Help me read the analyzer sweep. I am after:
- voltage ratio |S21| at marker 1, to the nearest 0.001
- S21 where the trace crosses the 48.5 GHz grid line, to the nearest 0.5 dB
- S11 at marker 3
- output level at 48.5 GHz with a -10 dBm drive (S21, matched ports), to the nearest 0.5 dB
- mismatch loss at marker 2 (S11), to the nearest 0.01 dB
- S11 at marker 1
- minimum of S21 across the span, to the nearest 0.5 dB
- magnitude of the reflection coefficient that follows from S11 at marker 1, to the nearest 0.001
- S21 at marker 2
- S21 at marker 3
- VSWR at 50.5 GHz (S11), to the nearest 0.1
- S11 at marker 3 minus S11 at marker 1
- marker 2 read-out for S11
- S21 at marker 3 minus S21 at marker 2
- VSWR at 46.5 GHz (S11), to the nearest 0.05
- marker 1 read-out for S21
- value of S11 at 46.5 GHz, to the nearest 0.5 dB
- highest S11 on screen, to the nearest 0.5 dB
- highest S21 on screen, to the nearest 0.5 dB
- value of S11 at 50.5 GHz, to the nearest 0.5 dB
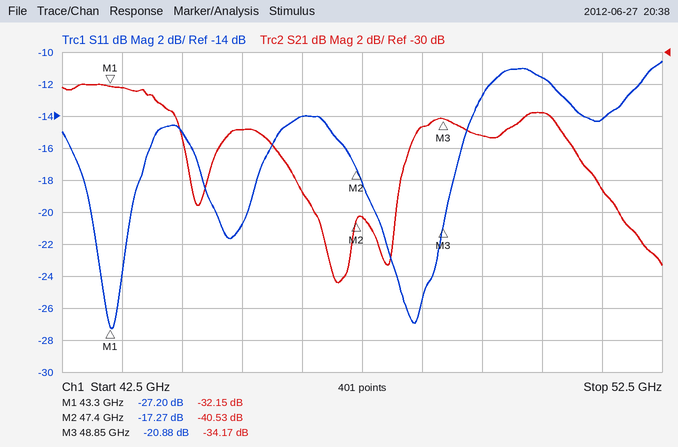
0.025
-34.5 dB
-20.88 dB
-44.5 dBm
0.08 dB
-27.20 dB
-44.5 dB
0.044
-40.53 dB
-34.17 dB
1.7
6.32 dB
-17.27 dB
6.36 dB
1.50
-32.15 dB
-14.0 dB
-10.5 dB
-32.0 dB
-11.5 dB
